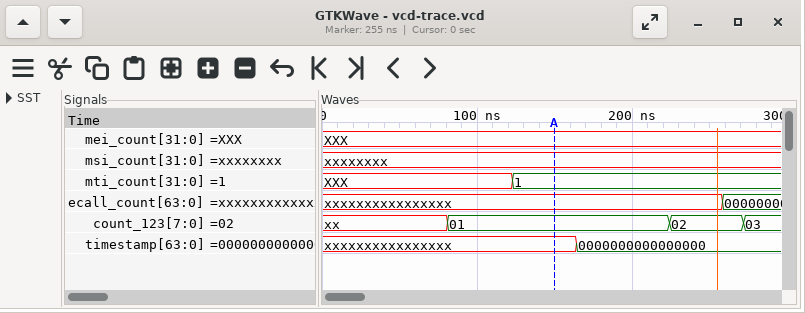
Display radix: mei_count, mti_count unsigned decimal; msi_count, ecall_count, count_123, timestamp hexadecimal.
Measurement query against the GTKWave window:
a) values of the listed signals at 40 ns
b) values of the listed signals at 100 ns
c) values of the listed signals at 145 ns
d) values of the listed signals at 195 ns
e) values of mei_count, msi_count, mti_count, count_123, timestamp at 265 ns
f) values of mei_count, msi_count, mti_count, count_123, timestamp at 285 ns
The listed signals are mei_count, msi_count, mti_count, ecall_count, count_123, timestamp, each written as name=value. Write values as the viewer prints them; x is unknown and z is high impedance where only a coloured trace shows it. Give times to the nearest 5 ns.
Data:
mei_count=XXX, msi_count=xxxxxxxx, mti_count=XXX, ecall_count=xxxxxxxxxxxxxxxx, count_123=xx, timestamp=xxxxxxxxxxxxxxxx
mei_count=XXX, msi_count=xxxxxxxx, mti_count=XXX, ecall_count=xxxxxxxxxxxxxxxx, count_123=01, timestamp=xxxxxxxxxxxxxxxx
mei_count=XXX, msi_count=xxxxxxxx, mti_count=1, ecall_count=xxxxxxxxxxxxxxxx, count_123=01, timestamp=xxxxxxxxxxxxxxxx
mei_count=XXX, msi_count=xxxxxxxx, mti_count=1, ecall_count=xxxxxxxxxxxxxxxx, count_123=01, timestamp=0000000000000000
mei_count=XXX, msi_count=xxxxxxxx, mti_count=1, count_123=02, timestamp=0000000000000000
mei_count=XXX, msi_count=xxxxxxxx, mti_count=1, count_123=03, timestamp=0000000000000000
